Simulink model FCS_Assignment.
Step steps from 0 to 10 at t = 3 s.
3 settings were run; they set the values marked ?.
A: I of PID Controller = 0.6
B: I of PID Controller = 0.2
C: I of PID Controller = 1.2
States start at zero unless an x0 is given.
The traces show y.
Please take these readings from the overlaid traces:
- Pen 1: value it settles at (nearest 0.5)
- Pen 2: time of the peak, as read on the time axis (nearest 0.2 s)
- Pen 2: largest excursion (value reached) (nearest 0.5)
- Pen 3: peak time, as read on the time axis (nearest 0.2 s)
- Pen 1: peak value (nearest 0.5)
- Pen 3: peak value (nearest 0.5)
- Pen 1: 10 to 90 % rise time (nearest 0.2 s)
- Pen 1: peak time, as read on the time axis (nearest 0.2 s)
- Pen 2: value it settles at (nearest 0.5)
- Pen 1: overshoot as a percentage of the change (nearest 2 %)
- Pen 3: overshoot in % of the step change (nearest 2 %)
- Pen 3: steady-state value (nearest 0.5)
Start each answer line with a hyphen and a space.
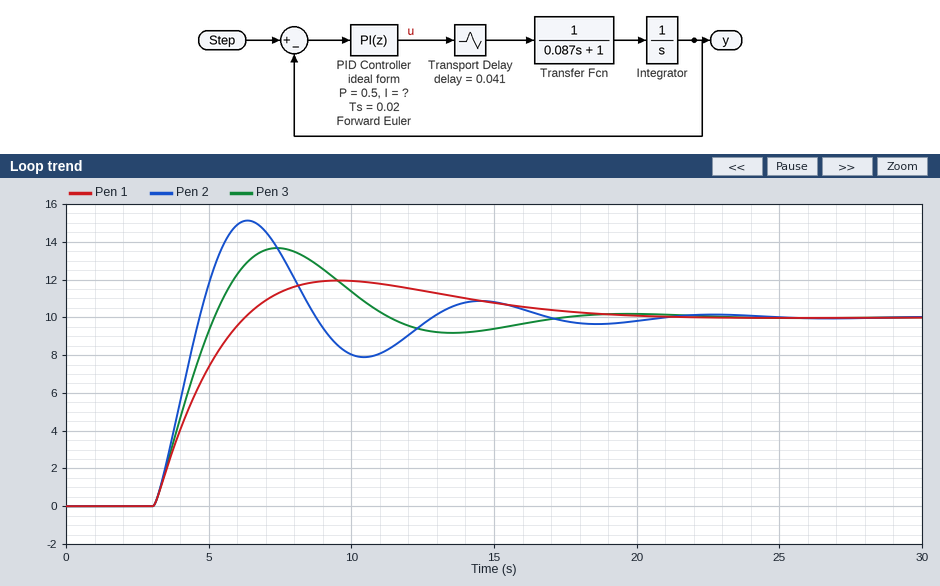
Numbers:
- 10.0
- 6.4 s
- 15.0
- 7.4 s
- 12.0
- 13.5
- 2.4 s
- 9.6 s
- 10.0
- 20 %
- 36 %
- 10.0
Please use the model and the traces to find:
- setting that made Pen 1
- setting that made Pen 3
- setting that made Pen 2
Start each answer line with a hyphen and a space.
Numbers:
- B
- A
- C
